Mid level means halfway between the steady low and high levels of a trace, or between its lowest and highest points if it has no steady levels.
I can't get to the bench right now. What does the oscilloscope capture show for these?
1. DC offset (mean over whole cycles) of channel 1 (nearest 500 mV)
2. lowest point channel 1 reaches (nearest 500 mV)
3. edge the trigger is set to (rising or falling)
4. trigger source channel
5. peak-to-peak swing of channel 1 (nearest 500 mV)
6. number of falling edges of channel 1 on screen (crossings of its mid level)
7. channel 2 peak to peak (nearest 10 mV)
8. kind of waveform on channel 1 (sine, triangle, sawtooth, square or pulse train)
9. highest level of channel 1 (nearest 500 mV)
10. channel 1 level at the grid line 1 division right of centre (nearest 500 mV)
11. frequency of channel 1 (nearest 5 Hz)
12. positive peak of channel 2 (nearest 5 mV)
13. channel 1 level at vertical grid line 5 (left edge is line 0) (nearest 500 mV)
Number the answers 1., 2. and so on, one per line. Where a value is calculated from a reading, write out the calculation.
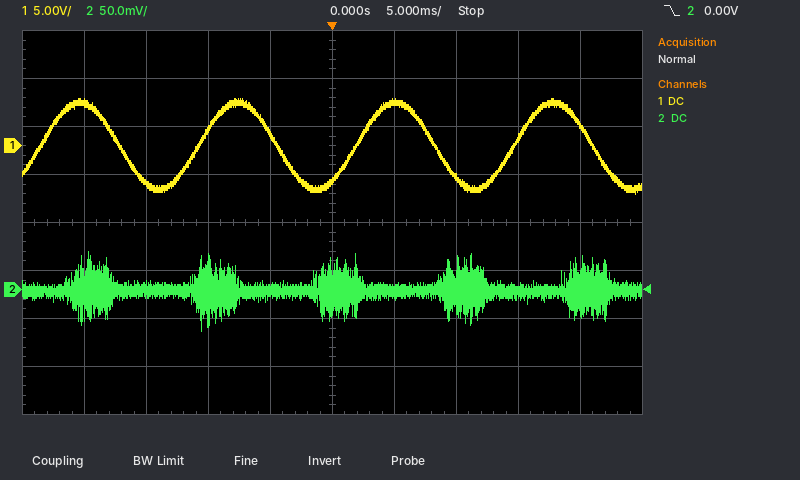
1. (5.0 V + (-5.0 V)) / 2 ≈ 0.0 V
2. -5.0 V
3. falling
4. channel 2
5. 5.0 V − (-5.0 V) = 10.0 V
6. 4
7. 80 mV
8. sine
9. 5.0 V
10. 4.5 V
11. 80 Hz
12. 40 mV
13. -3.5 V
